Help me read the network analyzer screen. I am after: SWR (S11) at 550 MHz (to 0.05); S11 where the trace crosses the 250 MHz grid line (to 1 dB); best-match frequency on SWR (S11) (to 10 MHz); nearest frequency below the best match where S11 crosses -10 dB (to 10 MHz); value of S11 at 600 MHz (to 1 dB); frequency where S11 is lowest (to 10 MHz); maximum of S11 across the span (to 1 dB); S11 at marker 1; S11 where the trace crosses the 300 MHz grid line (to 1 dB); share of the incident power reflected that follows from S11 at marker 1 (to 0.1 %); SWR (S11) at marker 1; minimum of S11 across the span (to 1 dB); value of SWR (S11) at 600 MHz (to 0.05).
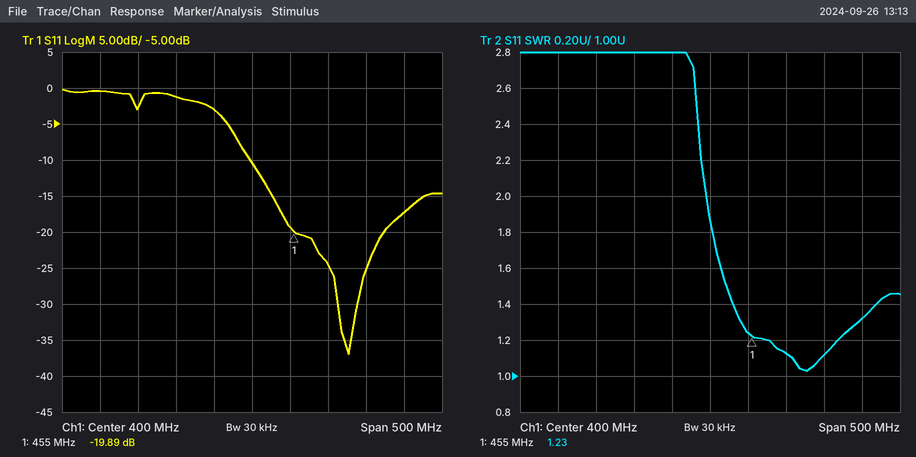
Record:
1.10
-3 dB
530 MHz
400 MHz
-17 dB
530 MHz
0 dB
-19.89 dB
-1 dB
1.0 %
1.23
-37 dB
1.30
